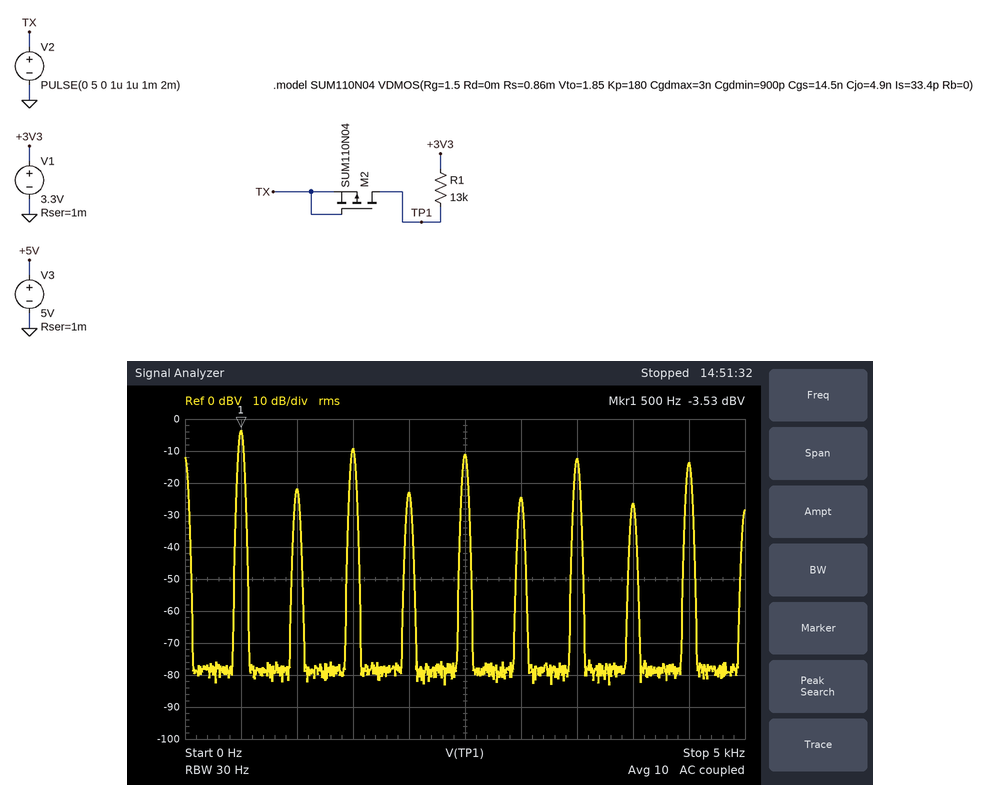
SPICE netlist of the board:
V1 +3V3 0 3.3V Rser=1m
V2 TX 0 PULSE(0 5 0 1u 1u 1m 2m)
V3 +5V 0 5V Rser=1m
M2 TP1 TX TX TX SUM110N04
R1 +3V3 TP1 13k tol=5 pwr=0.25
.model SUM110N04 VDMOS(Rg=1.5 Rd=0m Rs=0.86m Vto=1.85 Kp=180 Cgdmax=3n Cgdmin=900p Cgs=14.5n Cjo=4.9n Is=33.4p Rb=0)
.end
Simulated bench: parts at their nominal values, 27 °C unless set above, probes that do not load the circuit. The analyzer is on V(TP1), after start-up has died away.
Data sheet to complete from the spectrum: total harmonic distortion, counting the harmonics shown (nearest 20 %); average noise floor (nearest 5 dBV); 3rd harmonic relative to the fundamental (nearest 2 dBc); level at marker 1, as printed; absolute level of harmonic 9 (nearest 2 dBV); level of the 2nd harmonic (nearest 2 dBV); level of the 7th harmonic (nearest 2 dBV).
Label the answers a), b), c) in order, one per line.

a) 80 %
b) -80 dBV
c) -6 dBc
d) -3.53 dBV
e) -14 dBV
f) -22 dBV
g) -12 dBV
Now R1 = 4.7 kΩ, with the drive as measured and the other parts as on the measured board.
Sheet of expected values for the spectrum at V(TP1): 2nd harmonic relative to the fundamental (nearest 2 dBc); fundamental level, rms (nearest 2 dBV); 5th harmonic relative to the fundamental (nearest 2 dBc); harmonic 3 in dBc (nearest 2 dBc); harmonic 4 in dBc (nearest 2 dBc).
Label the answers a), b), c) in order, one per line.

a) -26 dBc
b) -4 dBV
c) -12 dBc
d) -8 dBc
e) -26 dBc
